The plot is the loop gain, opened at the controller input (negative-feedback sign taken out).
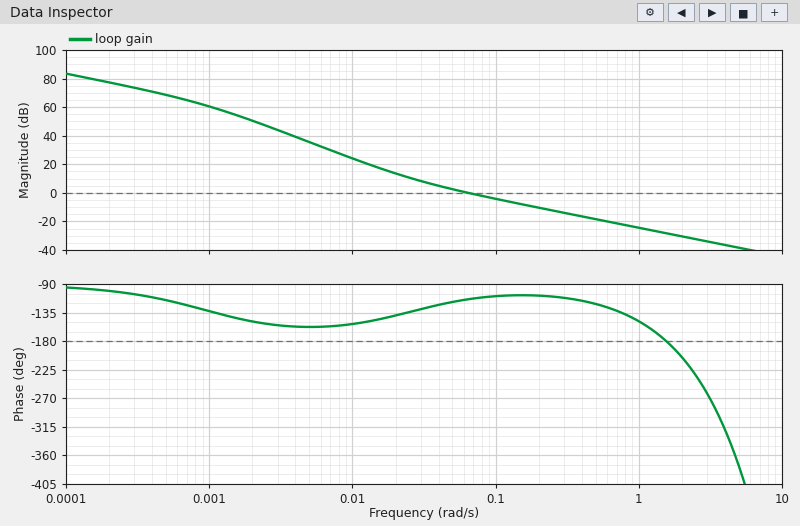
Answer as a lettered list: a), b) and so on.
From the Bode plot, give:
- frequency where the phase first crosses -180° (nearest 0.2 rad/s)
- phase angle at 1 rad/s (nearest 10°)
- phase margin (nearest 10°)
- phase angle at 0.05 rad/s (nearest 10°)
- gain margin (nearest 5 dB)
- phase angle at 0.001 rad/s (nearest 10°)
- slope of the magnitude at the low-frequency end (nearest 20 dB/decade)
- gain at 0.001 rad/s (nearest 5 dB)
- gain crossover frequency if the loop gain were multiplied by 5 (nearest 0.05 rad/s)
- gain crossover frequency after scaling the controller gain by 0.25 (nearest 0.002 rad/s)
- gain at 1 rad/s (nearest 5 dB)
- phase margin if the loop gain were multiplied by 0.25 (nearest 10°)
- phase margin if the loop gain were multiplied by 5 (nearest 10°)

a) 1.6 rad/s
b) -150°
c) 70°
d) -120°
e) 30 dB
f) -130°
g) -20 dB/decade
h) 60 dB
i) 0.30 rad/s
j) 0.022 rad/s
k) -25 dB
l) 40°
m) 70°
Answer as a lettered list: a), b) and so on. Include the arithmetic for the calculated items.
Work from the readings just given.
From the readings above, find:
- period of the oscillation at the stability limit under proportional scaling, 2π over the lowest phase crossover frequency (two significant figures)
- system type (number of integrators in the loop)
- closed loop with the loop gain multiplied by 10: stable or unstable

a) 2π / 1.6 = 3.9 s
b) 1
c) stable
